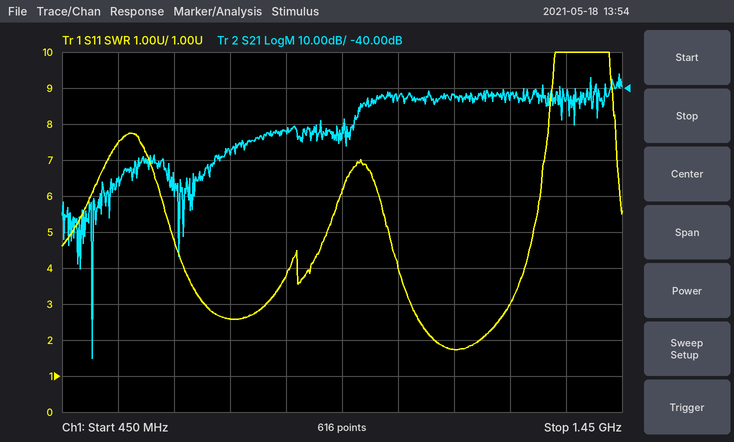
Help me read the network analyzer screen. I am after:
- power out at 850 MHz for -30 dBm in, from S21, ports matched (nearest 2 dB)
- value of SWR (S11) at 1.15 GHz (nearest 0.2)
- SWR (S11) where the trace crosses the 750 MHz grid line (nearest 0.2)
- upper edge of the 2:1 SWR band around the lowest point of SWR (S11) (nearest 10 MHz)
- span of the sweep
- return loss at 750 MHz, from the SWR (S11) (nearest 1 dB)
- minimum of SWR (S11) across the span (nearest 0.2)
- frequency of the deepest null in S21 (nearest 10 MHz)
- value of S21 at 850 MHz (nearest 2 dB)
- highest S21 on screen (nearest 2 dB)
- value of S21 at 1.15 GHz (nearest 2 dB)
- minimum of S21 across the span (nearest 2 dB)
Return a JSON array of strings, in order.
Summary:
["-82 dBm", "1.8", "2.6", "1.20 GHz", "1 GHz", "7 dB", "1.8", "500 MHz", "-52 dB", "-36 dB", "-42 dB", "-116 dB"]
